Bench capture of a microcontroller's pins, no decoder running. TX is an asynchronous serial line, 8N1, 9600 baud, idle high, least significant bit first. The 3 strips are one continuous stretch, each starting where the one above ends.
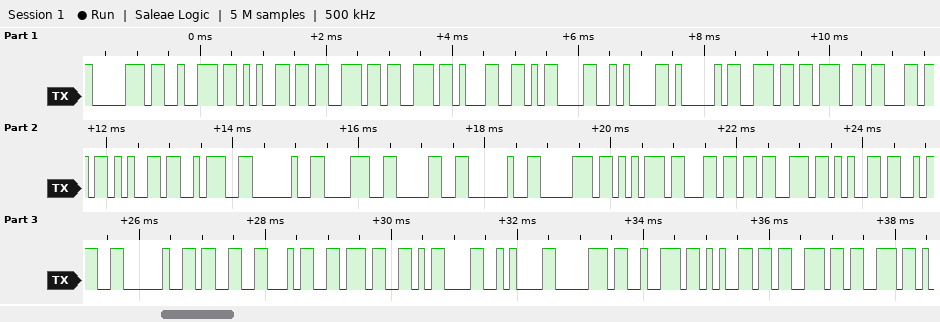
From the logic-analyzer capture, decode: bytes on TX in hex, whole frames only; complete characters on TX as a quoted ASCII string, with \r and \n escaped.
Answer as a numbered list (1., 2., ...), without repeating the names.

1. 70 72 65 73 73 31 0D 0A 41 6E 67 6C 65 3A 20 38 30 20 70 75 6C 73 65 3A 20 33 34 37 0D 0A 70 72 65 73 73
2. "press1\r\nAngle: 80 pulse: 347\r\npress"
